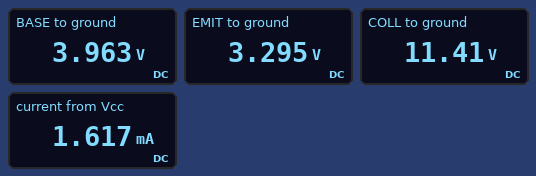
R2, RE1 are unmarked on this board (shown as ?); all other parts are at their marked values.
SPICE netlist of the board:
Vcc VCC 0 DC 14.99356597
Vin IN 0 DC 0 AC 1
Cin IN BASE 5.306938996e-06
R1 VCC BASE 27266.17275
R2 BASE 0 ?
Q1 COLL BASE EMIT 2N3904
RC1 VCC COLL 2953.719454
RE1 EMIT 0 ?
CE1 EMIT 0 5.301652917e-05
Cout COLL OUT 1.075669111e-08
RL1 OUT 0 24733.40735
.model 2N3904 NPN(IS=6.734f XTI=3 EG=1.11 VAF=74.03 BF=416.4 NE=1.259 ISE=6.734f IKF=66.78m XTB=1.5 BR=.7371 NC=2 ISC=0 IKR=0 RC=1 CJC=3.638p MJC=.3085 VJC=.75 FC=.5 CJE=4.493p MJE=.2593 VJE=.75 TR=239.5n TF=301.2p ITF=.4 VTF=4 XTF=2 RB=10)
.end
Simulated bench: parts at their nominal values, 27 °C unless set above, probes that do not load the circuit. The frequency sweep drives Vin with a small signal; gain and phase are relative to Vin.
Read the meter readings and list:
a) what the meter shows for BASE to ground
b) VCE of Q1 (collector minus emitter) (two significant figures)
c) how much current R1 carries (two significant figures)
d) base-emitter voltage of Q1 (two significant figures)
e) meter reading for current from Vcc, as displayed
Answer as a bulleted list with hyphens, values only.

- 3.963 V
- 8.1 V
- 400 µA
- 670 mV
- 1.617 mA
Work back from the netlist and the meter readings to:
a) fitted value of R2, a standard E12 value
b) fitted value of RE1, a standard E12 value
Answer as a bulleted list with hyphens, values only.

- 10 kΩ
- 2.7 kΩ
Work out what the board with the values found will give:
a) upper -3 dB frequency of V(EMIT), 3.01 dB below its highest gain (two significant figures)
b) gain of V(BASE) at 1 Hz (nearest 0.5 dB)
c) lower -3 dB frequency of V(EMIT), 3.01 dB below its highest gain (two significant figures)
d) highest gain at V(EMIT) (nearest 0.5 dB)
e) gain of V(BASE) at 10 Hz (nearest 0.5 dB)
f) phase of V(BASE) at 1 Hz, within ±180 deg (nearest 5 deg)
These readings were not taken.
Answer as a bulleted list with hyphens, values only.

- 150 Hz
- -12.5 dB
- 3.7 Hz
- -1.0 dB
- -1.0 dB
- 75 deg
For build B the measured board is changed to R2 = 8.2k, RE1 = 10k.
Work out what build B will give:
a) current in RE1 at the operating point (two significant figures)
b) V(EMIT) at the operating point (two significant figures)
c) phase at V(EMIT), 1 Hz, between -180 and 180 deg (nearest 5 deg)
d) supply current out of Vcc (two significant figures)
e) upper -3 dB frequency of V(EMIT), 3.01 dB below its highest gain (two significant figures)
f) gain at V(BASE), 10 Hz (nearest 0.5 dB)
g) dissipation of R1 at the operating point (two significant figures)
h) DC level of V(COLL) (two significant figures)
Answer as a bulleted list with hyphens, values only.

- 280 µA
- 2.8 V
- 75 deg
- 700 µA
- 43 Hz
- -1.5 dB
- 4.9 mW
- 14 V
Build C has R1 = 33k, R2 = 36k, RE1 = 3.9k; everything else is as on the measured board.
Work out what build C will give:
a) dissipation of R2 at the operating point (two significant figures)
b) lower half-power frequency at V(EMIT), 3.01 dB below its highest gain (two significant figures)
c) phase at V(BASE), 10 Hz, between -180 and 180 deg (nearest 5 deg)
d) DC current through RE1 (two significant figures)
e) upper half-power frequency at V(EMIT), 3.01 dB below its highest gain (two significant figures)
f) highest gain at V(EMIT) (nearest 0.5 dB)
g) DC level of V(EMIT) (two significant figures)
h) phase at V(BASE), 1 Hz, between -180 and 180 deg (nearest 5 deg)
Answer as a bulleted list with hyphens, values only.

- 1.6 mW
- 1.7 Hz
- 10 deg
- 1.8 mA
- 200 Hz
- -0.5 dB
- 6.9 V
- 60 deg
